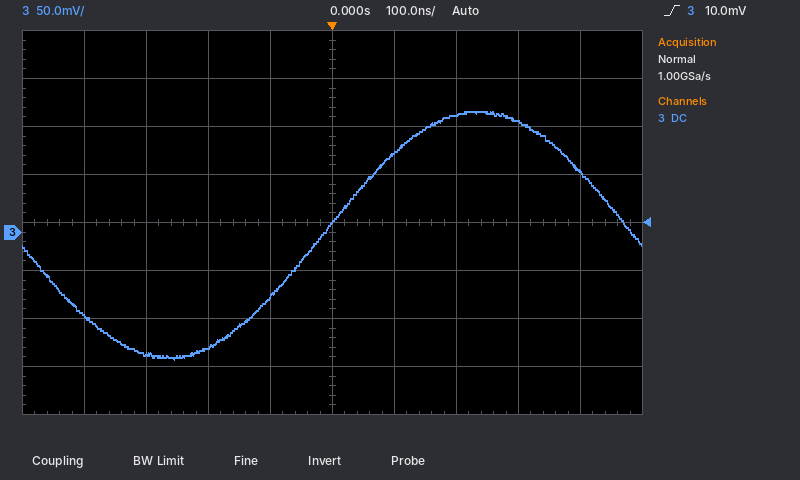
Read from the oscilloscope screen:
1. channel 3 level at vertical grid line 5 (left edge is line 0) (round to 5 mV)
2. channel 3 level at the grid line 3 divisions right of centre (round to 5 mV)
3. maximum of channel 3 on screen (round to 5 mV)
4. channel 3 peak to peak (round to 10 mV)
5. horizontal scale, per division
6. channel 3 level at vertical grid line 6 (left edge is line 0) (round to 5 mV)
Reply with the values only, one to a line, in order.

10 mV
115 mV
125 mV
260 mV
100 ns
80 mV
